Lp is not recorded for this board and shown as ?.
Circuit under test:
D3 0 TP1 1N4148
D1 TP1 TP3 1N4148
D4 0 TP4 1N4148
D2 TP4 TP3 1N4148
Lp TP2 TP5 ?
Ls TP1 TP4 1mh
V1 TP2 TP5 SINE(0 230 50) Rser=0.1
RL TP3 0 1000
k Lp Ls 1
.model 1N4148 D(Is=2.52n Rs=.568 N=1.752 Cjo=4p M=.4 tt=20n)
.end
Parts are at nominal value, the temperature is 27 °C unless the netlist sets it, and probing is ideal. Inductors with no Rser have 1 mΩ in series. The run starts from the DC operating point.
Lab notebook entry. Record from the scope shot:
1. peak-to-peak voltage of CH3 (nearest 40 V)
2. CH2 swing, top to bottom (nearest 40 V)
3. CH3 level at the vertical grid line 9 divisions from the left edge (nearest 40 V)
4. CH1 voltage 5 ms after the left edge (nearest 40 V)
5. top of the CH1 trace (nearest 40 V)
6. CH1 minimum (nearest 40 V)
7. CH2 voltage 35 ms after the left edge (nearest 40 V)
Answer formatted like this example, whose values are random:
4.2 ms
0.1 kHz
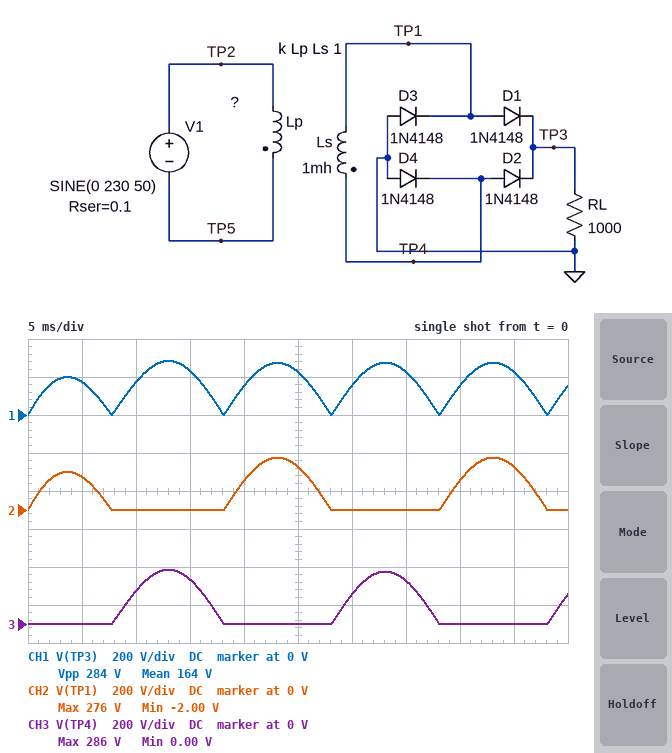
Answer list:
280 V
280 V
0 V
160 V
280 V
0 V
0 V
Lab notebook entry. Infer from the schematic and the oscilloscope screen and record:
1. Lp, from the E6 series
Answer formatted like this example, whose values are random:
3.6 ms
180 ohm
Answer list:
470 µH
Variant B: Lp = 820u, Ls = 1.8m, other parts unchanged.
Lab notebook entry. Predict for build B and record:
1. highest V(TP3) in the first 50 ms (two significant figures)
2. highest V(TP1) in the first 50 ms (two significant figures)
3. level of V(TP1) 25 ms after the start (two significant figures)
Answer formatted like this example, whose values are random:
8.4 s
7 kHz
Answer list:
340 V
320 V
290 V
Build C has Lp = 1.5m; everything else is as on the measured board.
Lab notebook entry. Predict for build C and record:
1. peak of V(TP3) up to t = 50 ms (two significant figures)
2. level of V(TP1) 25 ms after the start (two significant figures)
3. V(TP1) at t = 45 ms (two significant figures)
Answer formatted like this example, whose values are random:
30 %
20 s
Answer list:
200 V
170 V
180 V
